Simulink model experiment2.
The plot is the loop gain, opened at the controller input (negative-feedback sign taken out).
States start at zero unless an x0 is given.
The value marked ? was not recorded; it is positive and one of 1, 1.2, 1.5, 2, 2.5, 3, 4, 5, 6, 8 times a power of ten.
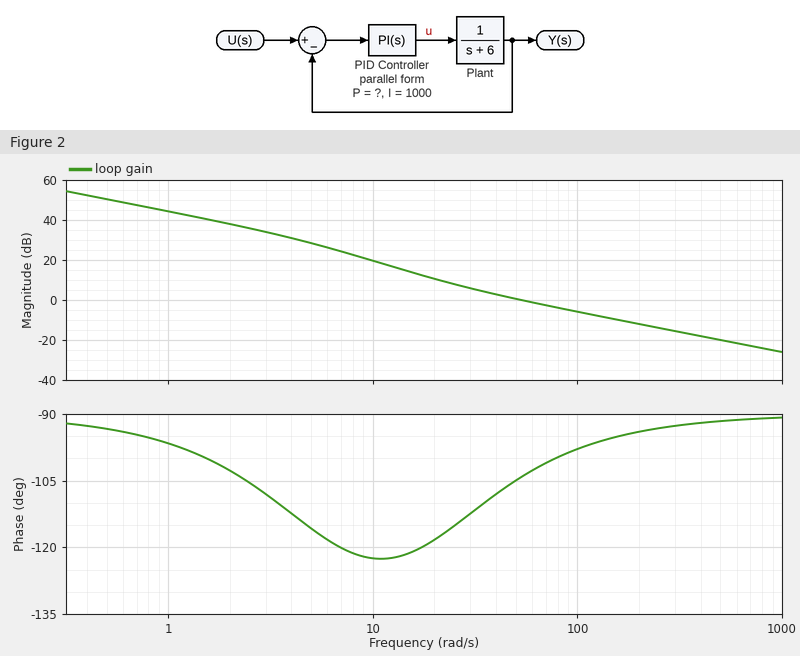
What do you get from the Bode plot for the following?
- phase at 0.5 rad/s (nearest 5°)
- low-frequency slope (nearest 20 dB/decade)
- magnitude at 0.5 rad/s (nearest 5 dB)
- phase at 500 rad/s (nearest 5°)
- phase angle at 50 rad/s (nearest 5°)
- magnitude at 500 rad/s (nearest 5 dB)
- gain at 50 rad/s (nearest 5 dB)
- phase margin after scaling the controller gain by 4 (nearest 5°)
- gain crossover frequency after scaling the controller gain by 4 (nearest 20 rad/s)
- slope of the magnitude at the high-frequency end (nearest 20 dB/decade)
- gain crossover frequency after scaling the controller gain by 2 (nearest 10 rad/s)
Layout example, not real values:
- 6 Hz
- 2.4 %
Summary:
- -95°
- -20 dB/decade
- 50 dB
- -90°
- -105°
- -20 dB
- 0 dB
- 85°
- 200 rad/s
- -20 dB/decade
- 100 rad/s
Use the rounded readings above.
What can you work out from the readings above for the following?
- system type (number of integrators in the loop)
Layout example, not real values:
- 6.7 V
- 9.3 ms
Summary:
- 1
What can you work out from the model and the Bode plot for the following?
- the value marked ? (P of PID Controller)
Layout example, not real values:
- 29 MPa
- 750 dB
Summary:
- 50
